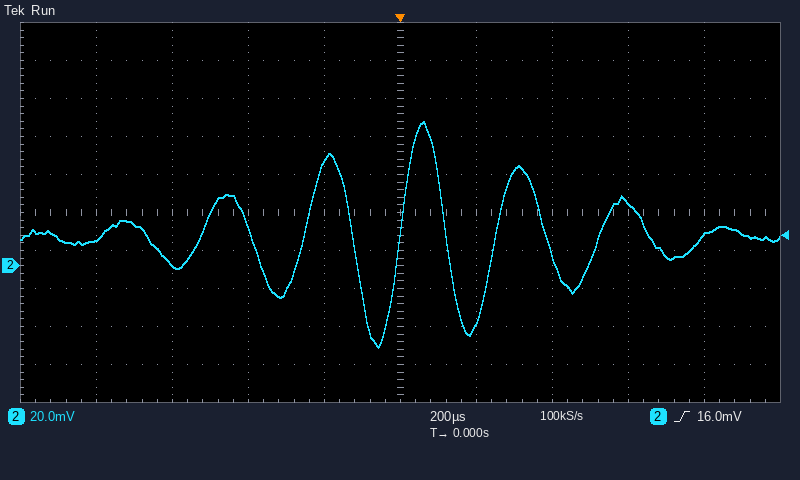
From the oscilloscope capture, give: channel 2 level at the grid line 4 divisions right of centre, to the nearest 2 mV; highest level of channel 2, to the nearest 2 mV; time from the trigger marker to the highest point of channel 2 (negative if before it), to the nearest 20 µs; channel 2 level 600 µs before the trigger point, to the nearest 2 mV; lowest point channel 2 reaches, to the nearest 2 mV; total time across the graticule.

16 mV
76 mV
+60 µs
0 mV
-44 mV
2 ms
